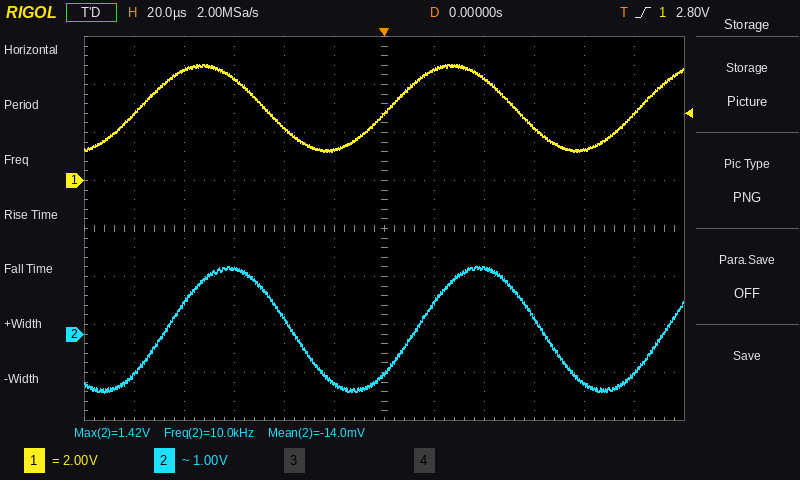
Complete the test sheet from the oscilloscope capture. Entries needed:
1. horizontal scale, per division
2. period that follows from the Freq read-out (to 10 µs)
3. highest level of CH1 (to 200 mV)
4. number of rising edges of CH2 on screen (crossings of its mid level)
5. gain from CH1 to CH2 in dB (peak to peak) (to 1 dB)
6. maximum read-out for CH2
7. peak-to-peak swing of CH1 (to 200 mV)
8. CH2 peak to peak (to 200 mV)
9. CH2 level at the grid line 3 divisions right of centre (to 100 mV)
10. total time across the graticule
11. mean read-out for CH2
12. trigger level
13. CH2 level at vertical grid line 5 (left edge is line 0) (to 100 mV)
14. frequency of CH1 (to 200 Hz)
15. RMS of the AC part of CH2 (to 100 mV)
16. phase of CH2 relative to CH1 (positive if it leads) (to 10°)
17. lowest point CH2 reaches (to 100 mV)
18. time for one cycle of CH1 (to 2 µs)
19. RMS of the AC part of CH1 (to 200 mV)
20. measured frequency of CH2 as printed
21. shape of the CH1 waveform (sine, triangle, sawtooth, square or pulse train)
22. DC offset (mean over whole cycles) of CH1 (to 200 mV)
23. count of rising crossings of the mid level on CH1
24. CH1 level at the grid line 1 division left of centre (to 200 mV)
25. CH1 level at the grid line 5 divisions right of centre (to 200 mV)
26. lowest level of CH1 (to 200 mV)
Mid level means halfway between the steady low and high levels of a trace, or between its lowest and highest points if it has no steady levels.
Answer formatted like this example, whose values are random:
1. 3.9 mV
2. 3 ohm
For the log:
1. 20 µs
2. 100 µs
3. 4.8 V
4. 3
5. -3 dB
6. 1.42 V
7. 3.6 V
8. 2.6 V
9. 300 mV
10. 240 µs
11. -14.0 mV
12. 2.80 V
13. -1.0 V
14. 10.0 kHz
15. 900 mV
16. -40°
17. -1.2 V
18. 100 µs
19. 1.2 V
20. 10.0 kHz
21. sine
22. 3.0 V
23. 3
24. 1.2 V
25. 2.8 V
26. 1.2 V
